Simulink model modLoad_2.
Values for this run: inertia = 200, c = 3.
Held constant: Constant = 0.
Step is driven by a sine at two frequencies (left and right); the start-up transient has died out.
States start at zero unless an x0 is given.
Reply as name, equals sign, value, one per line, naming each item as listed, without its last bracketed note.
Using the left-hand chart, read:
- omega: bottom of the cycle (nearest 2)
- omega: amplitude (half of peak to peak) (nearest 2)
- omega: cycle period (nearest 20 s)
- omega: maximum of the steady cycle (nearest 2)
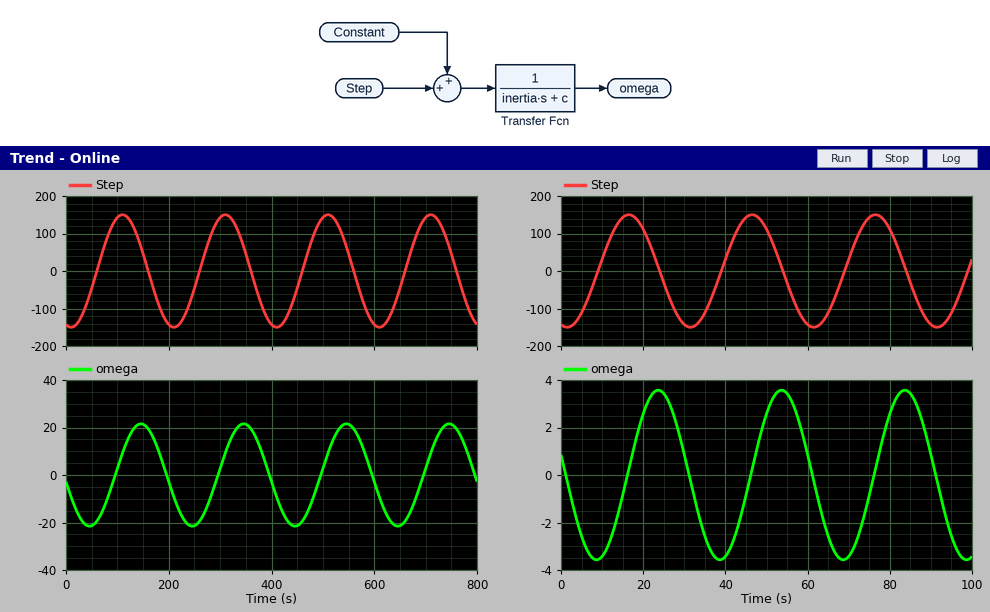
omega: bottom of the cycle = -22
omega: amplitude (half of peak to peak) = 22
omega: cycle period = 200 s
omega: maximum of the steady cycle = 22
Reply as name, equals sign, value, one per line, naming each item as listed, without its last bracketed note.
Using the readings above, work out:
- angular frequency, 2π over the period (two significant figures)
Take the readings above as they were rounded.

angular frequency, 2π over the period = 0.031 rad/s
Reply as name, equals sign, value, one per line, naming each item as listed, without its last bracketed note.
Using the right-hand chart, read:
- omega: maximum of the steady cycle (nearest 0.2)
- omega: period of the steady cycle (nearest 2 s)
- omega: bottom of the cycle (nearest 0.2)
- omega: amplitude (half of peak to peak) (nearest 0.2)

omega: maximum of the steady cycle = 3.6
omega: period of the steady cycle = 30 s
omega: bottom of the cycle = -3.6
omega: amplitude (half of peak to peak) = 3.6
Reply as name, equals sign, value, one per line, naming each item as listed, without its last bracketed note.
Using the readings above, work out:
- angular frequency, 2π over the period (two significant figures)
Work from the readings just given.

angular frequency, 2π over the period = 0.21 rad/s
